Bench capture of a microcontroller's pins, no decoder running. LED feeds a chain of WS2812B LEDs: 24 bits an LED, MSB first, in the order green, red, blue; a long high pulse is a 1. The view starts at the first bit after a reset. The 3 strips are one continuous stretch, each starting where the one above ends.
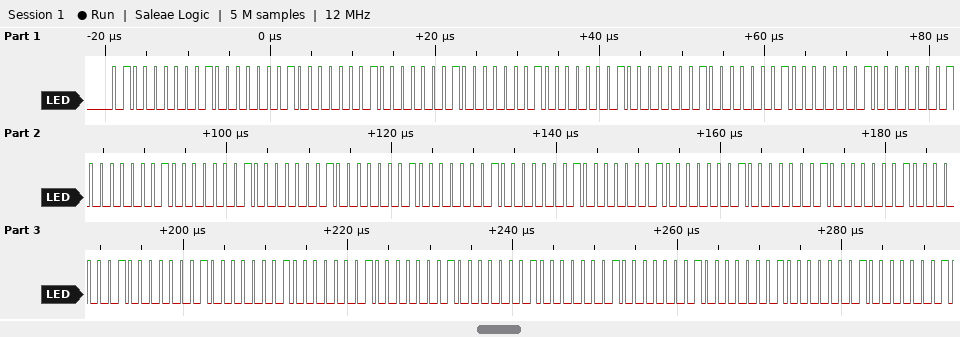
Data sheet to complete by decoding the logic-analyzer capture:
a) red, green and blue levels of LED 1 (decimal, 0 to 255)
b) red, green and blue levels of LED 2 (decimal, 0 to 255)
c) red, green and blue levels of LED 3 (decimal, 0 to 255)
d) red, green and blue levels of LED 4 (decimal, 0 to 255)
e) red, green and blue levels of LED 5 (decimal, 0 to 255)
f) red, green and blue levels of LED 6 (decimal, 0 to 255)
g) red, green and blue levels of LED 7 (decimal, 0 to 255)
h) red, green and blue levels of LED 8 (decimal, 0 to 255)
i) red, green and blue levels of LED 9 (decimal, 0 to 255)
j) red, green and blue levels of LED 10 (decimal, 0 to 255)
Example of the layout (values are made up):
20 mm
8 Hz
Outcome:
64, 64, 64
64, 64, 64
64, 64, 64
64, 64, 64
64, 64, 64
64, 64, 64
64, 64, 64
64, 64, 64
64, 64, 64
64, 64, 64
